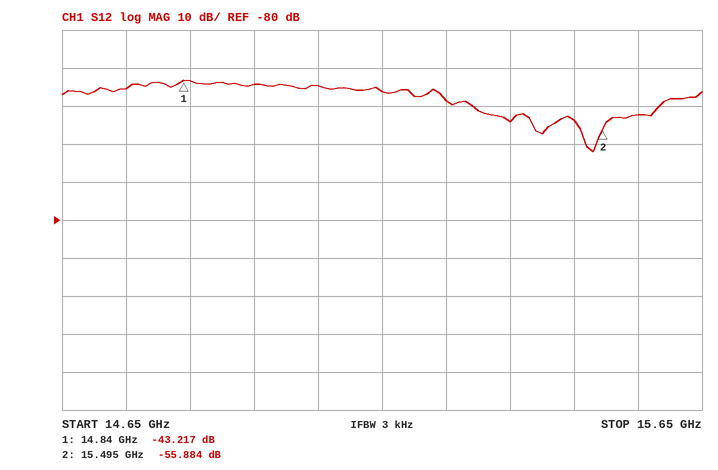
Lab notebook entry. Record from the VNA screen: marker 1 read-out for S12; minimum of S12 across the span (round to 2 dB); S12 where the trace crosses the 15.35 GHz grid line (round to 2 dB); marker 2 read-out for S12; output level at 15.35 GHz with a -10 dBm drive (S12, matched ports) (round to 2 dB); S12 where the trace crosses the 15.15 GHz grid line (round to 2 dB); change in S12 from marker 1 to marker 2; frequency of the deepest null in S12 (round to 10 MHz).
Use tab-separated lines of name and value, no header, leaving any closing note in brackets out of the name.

marker 1 read-out for S12	-43.217 dB
minimum of S12 across the span	-62 dB
S12 where the trace crosses the 15.35 GHz grid line	-54 dB
marker 2 read-out for S12	-55.884 dB
output level at 15.35 GHz with a -10 dBm drive (S12, matched ports)	-64 dBm
S12 where the trace crosses the 15.15 GHz grid line	-46 dB
change in S12 from marker 1 to marker 2	-12.667 dB
frequency of the deepest null in S12	15.48 GHz
